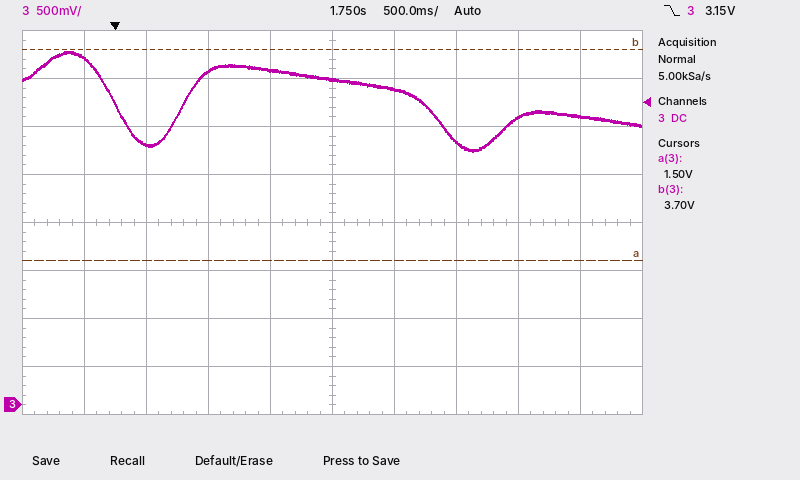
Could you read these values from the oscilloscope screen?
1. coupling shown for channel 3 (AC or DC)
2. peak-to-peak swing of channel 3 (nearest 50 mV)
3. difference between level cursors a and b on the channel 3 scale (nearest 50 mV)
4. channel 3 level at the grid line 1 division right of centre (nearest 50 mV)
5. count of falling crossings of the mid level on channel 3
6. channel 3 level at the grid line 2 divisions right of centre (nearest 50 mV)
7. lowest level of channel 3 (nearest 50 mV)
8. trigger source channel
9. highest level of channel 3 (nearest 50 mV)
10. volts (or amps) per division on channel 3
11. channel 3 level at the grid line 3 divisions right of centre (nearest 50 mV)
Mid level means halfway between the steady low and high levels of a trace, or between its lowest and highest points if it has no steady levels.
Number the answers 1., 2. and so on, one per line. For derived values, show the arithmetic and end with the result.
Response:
1. DC
2. 3.70 V − (2.65 V) = 1.05 V
3. 2.20 V
4. 3.30 V
5. 2
6. 2.75 V
7. 2.65 V
8. channel 3
9. 3.70 V
10. 500 mV
11. 3.00 V
